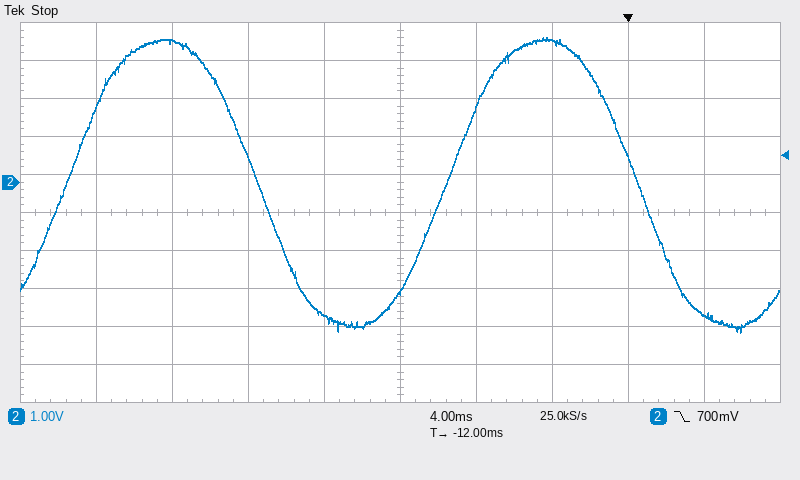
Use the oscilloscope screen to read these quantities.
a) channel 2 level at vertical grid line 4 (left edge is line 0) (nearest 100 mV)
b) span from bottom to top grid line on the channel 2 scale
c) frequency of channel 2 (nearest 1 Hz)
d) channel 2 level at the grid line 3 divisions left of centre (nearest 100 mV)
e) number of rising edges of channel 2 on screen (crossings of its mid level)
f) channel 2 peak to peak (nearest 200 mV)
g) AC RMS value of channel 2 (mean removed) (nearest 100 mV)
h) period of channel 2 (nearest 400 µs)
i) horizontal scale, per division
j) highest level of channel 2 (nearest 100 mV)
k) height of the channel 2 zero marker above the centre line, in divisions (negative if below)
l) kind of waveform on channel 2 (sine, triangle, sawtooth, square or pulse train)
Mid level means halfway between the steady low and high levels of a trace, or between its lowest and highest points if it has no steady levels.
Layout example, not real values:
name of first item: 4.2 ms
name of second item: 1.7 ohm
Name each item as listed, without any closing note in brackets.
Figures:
channel 2 level at vertical grid line 4 (left edge is line 0): -3.5 V
span from bottom to top grid line on the channel 2 scale: 10 V
frequency of channel 2: 50 Hz
channel 2 level at the grid line 3 divisions left of centre: 3.7 V
number of rising edges of channel 2 on screen: 2
channel 2 peak to peak: 7.8 V
AC RMS value of channel 2 (mean removed): 2.8 V
period of channel 2: 20.0 ms
horizontal scale, per division: 4 ms
highest level of channel 2: 3.8 V
height of the channel 2 zero marker above the centre line, in divisions: +0.8 div
kind of waveform on channel 2: sine
